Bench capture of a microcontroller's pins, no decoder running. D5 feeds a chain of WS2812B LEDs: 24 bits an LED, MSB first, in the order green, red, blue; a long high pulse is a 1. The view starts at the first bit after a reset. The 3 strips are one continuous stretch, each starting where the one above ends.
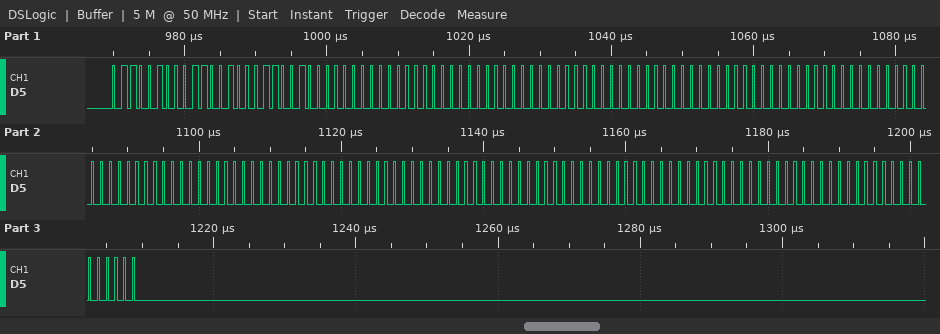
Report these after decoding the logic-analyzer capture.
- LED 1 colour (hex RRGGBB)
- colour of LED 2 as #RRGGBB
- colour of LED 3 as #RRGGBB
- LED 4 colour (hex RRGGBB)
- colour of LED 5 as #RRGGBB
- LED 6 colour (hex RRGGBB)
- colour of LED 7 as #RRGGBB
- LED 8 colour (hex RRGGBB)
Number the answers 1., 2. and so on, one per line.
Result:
1. #646464
2. #000000
3. #000000
4. #000000
5. #000000
6. #000000
7. #000000
8. #000000
